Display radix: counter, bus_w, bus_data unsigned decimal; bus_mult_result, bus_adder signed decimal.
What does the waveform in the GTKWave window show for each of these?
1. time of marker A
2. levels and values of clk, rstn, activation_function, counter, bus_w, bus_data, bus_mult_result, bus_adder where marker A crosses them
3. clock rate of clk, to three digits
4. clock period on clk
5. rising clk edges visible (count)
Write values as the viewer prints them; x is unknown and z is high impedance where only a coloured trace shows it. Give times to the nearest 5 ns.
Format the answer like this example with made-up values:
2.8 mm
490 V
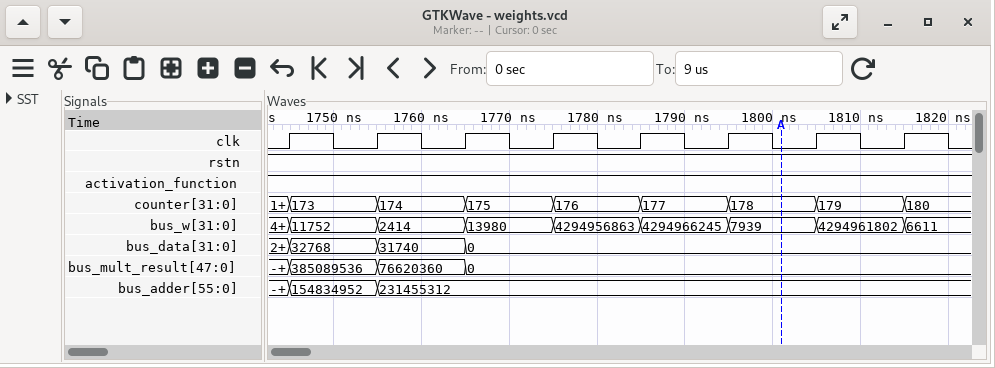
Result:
1800 ns
clk=0, rstn=1, activation_function=1, counter=178, bus_w=7939, bus_data=0, bus_mult_result=0, bus_adder=231455312
100 MHz
10 ns
8
